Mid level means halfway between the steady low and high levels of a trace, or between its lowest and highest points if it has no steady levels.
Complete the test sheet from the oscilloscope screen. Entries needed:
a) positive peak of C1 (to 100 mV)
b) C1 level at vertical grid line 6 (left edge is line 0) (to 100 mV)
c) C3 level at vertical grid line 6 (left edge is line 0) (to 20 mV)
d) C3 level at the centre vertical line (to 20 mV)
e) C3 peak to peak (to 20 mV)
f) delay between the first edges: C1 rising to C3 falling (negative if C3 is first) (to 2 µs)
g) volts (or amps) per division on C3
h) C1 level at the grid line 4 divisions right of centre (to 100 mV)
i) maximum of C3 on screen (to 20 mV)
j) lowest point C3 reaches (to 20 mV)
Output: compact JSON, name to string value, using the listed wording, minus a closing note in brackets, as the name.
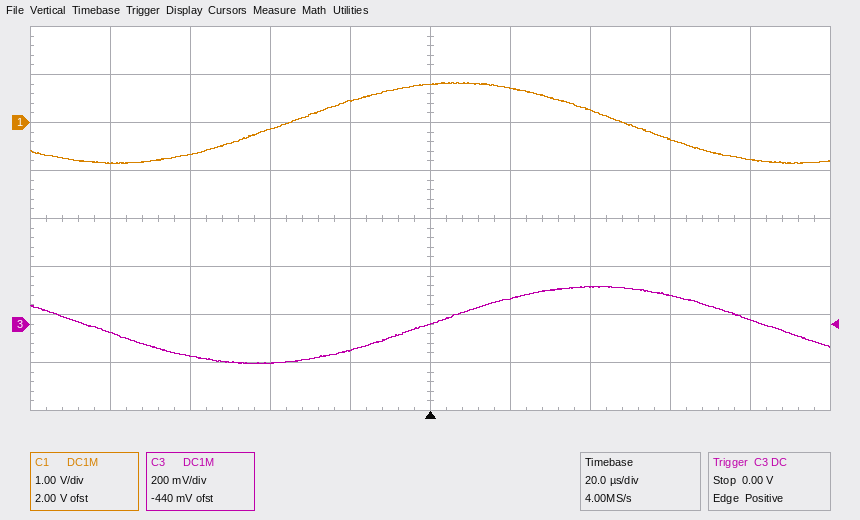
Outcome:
{"positive peak of C1": "800 mV", "C1 level at vertical grid line 6 (left edge is line 0)": "700 mV", "C3 level at vertical grid line 6 (left edge is line 0)": "100 mV", "C3 level at the centre vertical line": "0 mV", "C3 peak to peak": "320 mV", "delay between the first edges: C1 rising to C3 falling (negative if C3 is first)": "-50 µs", "volts (or amps) per division on C3": "200 mV", "C1 level at the grid line 4 divisions right of centre": "-800 mV", "maximum of C3 on screen": "160 mV", "lowest point C3 reaches": "-160 mV"}
